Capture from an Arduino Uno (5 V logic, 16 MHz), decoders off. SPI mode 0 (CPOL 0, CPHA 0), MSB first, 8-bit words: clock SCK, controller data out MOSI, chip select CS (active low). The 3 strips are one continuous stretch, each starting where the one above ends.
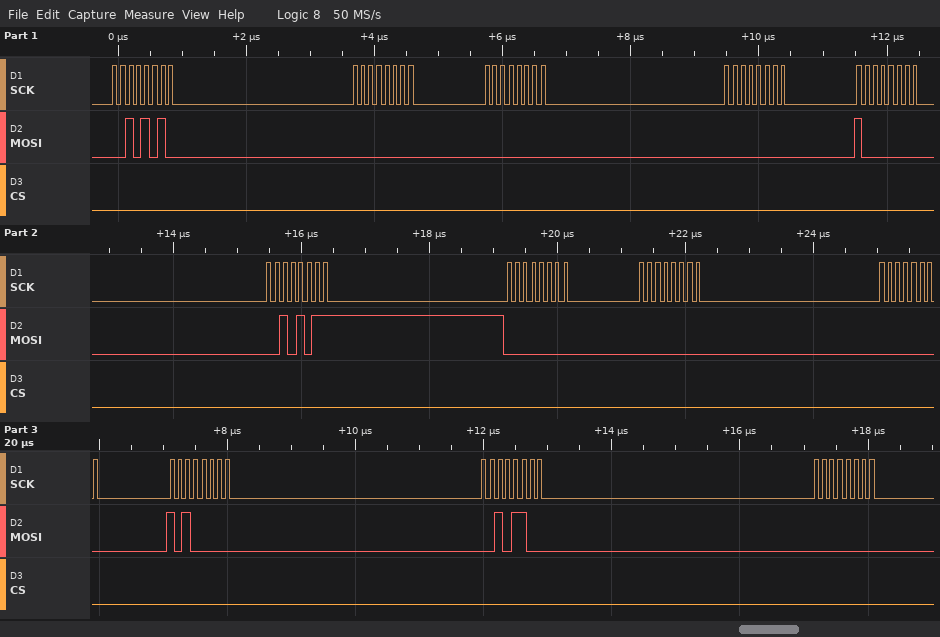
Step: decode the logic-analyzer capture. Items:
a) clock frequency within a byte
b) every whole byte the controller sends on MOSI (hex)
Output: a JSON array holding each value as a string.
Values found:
["8 MHz", "0x2A 0x00 0x00 0x00 0x80 0x2B 0x00 0x00 0x00 0xA0 0x2C 0x00"]
